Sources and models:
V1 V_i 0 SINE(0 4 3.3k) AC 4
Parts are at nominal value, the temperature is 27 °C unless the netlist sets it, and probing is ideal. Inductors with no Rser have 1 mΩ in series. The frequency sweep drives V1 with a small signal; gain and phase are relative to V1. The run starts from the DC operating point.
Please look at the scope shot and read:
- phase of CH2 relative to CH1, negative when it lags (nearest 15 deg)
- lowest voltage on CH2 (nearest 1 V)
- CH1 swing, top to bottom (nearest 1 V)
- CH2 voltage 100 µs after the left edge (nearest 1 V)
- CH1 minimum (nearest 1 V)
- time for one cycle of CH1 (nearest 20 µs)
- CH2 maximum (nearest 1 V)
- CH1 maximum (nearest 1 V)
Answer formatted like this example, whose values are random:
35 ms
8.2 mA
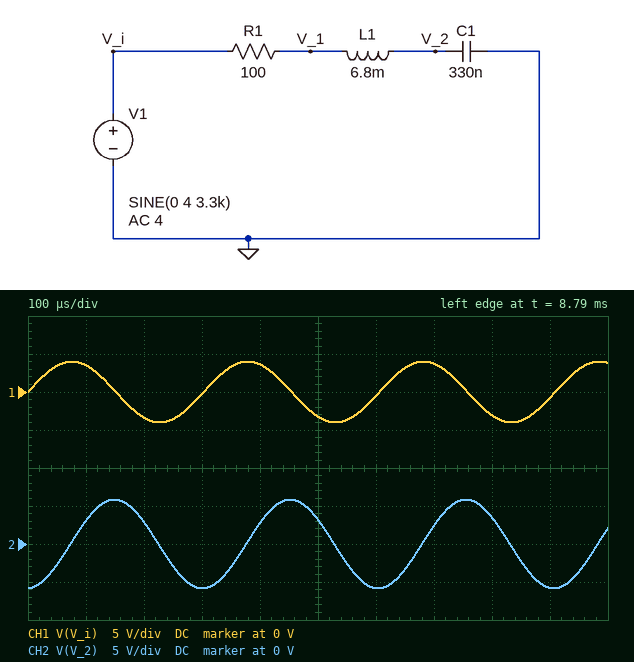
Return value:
-90 deg
-6 V
8 V
3 V
-4 V
300 µs
6 V
4 V
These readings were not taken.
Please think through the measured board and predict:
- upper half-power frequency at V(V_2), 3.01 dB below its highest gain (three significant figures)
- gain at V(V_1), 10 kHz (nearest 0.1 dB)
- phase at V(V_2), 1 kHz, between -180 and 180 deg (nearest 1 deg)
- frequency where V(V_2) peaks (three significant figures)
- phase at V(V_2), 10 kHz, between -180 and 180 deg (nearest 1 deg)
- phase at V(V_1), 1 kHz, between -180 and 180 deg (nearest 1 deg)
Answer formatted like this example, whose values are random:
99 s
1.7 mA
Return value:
3.99 kHz
-0.3 dB
-13 deg
2.92 kHz
-165 deg
-13 deg
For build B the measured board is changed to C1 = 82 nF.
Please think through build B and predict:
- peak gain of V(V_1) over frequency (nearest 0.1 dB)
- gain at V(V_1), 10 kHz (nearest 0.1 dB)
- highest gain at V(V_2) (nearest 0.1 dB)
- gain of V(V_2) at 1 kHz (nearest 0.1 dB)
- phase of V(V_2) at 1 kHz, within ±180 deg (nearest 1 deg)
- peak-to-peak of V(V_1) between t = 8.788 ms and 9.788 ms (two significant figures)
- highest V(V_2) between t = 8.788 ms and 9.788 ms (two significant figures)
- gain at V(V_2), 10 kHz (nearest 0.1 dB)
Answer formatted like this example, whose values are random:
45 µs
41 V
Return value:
0 dB
-0.7 dB
9.3 dB
0.2 dB
-3 deg
7.8 V
5.1 V
-2.3 dB
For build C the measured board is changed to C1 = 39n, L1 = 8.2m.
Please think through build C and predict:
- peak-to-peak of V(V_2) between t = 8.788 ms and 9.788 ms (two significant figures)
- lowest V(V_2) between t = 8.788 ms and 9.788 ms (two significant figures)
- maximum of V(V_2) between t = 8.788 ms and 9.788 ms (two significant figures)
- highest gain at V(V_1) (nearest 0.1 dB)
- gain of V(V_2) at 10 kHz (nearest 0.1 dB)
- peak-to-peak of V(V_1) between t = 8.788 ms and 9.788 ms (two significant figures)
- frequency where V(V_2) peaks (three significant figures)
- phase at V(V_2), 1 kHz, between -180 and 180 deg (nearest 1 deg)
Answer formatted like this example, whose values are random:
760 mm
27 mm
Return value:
9.2 V
-4.6 V
4.6 V
0 dB
8.9 dB
8.0 V
8.79 kHz
-1 deg
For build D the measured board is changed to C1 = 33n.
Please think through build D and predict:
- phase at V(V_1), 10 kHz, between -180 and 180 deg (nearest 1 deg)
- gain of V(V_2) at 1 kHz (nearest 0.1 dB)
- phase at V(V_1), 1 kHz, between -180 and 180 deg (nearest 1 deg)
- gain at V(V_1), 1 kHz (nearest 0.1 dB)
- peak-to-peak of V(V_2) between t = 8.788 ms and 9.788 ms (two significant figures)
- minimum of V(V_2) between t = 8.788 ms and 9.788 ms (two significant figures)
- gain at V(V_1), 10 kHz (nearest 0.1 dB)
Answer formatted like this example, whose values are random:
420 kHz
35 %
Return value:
-61 deg
0.1 dB
-1 deg
0 dB
8.8 V
-4.4 V
-6.3 dB
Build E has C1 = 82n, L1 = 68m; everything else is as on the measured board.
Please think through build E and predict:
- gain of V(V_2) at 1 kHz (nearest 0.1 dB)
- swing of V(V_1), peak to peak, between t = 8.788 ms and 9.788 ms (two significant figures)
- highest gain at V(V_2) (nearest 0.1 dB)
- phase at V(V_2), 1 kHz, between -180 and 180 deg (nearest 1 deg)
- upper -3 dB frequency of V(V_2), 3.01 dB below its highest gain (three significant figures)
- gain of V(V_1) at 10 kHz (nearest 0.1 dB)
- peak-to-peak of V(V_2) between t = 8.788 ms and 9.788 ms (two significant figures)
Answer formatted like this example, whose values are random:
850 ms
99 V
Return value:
2.1 dB
7.9 V
19.2 dB
-4 deg
2.24 kHz
0 dB
5.7 V
